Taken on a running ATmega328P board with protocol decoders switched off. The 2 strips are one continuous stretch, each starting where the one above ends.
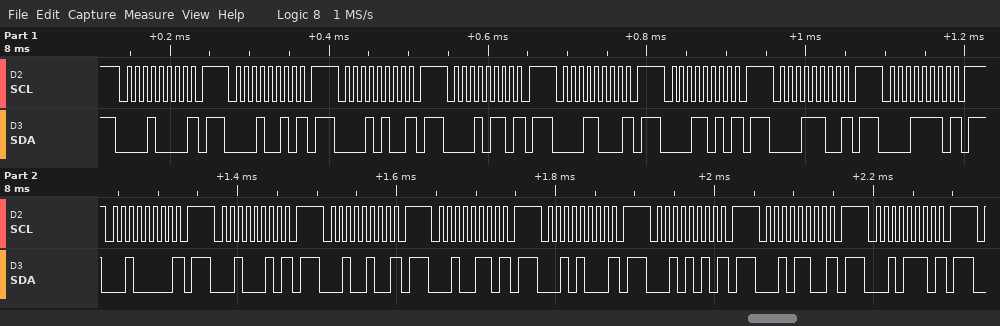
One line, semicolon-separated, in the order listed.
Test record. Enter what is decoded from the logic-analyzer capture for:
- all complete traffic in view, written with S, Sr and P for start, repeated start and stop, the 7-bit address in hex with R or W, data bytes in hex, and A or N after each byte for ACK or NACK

S 08W N P S 09W N P S 0AW N P S 0BW N P S 0CW N P S 0DW N P S 0EW N P S 0FW N P S 10W N P S 11W N P S 12W N P S 13W N P S 14W N P S 15W N P S 16W N P S 17W N P
